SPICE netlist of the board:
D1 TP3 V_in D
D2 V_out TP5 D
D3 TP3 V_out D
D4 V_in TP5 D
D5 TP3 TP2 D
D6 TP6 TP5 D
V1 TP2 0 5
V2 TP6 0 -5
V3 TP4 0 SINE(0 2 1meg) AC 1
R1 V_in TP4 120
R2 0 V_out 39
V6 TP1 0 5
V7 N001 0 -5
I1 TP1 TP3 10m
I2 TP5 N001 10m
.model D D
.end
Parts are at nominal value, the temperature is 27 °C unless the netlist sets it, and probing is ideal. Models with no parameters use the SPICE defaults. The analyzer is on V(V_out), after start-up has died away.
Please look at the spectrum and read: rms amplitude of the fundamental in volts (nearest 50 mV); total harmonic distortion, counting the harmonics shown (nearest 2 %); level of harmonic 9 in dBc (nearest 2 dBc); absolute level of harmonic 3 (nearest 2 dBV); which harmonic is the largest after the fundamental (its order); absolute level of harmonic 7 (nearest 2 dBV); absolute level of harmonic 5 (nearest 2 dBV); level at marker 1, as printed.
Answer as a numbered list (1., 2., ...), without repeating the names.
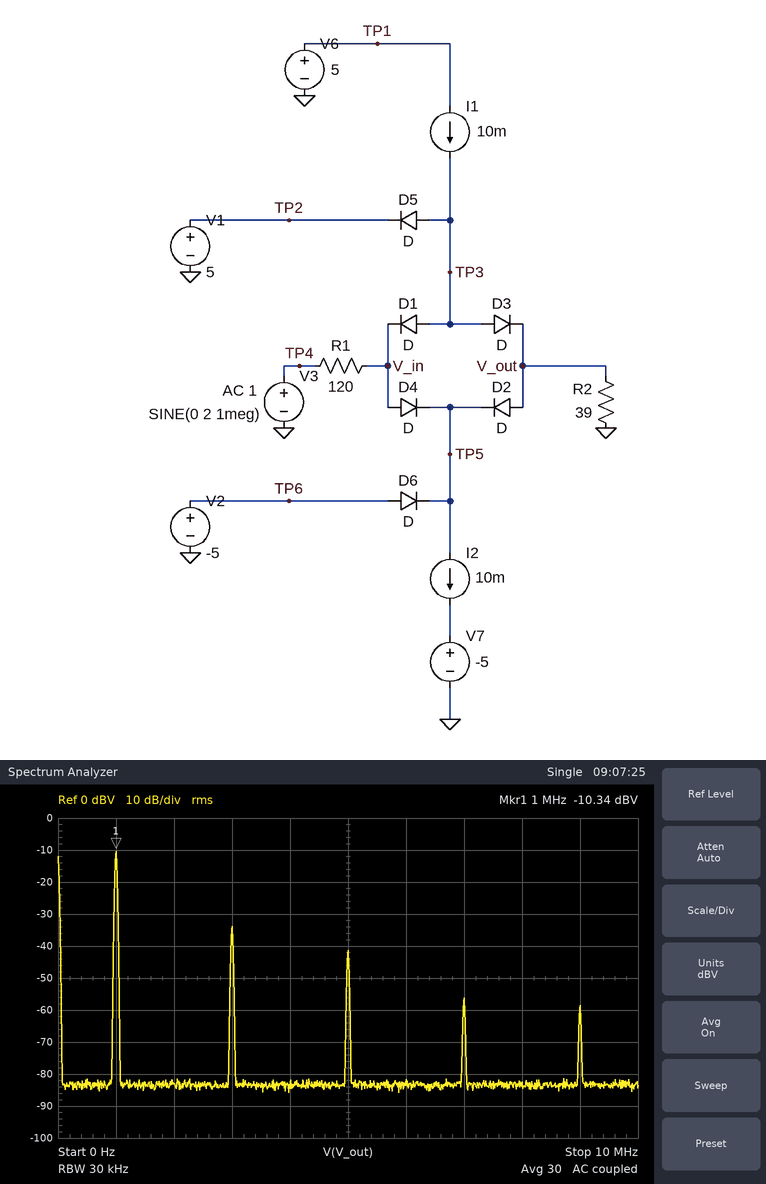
1. 300 mV
2. 8 %
3. -48 dBc
4. -34 dBV
5. 3
6. -56 dBV
7. -42 dBV
8. -10.34 dBV
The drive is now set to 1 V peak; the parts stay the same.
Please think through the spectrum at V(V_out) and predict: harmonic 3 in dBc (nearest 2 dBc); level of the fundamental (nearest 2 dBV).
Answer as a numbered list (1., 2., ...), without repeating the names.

1. -58 dBc
2. -16 dBV
